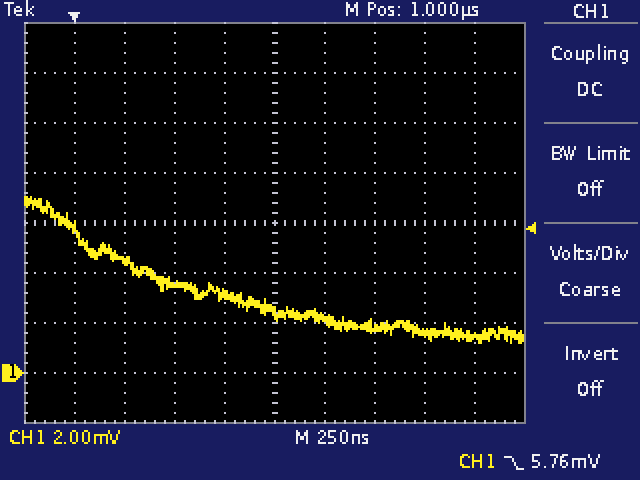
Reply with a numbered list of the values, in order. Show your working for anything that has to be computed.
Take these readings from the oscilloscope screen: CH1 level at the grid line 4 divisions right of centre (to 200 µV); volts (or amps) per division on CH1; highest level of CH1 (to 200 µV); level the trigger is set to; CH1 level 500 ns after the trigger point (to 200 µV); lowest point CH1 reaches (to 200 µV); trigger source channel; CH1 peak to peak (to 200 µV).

1. 1.4 mV
2. 2 mV
3. 7.0 mV
4. 5.76 mV
5. 3.6 mV
6. 1.2 mV
7. CH1
8. 7.0 mV − (1.2 mV) = 5.8 mV
